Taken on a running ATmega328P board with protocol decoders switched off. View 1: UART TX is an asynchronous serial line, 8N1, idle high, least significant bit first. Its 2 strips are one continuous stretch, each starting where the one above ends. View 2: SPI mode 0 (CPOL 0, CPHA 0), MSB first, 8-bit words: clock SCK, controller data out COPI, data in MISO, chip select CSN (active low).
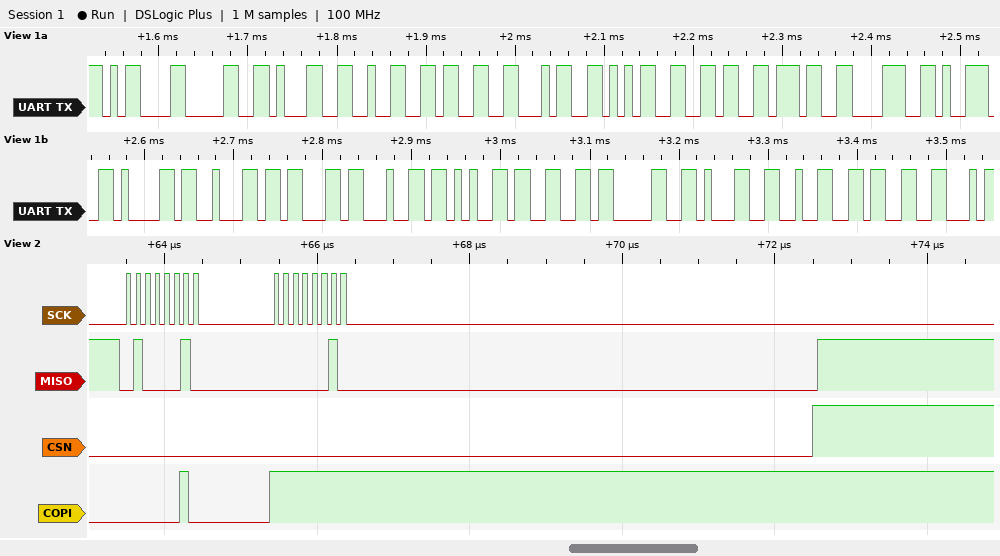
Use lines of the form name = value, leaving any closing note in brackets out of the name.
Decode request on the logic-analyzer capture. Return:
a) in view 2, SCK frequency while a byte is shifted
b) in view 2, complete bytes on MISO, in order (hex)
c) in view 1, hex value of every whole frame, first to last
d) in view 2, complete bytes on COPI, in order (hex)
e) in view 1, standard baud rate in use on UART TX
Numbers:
in view 2, SCK frequency while a byte is shifted = 8 MHz
in view 2, complete bytes on MISO, in order = 0x42 0x02
in view 1, hex value of every whole frame, first to last = 0D 30 31 32 33 34 35 36 37 38 39 61 62 63 64 65 66 30 31 32 33
in view 2, complete bytes on COPI, in order = 0x02 0xFF
in view 1, standard baud rate in use on UART TX = 115200 baud
